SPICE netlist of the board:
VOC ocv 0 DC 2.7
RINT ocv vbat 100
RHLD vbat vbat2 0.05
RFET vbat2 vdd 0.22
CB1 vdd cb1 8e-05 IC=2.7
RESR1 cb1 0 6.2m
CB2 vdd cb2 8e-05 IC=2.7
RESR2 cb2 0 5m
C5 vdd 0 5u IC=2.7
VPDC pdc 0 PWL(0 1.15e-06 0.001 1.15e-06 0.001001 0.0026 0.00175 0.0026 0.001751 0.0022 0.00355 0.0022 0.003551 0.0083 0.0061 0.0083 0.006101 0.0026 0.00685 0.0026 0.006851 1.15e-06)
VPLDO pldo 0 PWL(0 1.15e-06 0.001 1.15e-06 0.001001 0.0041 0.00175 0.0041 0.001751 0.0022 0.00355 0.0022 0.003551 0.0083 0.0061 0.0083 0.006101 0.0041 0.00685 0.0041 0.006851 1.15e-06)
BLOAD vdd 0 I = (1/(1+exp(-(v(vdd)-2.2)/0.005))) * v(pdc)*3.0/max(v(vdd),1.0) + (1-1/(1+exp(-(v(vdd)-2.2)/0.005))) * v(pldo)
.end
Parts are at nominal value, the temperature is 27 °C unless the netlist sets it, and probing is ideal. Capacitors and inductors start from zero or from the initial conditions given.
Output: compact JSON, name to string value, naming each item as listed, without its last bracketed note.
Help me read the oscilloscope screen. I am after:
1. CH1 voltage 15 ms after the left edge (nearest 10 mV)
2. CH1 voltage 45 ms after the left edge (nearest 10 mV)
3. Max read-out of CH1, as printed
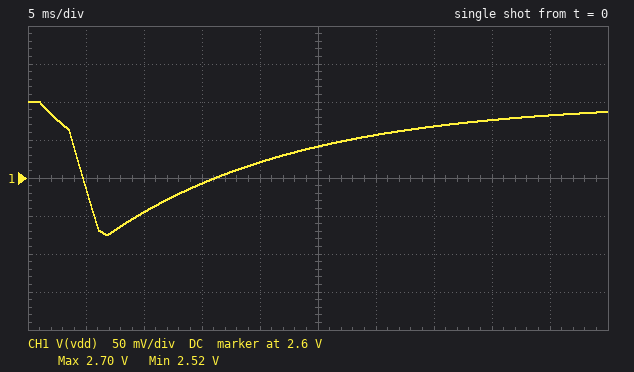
{"CH1 voltage 15 ms after the left edge": "2.59 V", "CH1 voltage 45 ms after the left edge": "2.68 V", "Max read-out of CH1, as printed": "2.70 V"}
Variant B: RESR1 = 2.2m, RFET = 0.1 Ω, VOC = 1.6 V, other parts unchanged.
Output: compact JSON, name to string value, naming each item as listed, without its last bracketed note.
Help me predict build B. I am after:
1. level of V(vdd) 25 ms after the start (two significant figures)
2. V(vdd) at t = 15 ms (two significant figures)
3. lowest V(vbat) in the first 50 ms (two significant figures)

{"level of V(vdd) 25 ms after the start": "1.8 V", "V(vdd) at t = 15 ms": "1.9 V", "lowest V(vbat) in the first 50 ms": "1.6 V"}
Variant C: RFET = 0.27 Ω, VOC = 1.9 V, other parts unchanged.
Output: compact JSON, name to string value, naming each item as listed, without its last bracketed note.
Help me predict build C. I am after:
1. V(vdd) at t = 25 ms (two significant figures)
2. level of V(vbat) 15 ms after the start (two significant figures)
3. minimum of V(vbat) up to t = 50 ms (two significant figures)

{"V(vdd) at t = 25 ms": "2.0 V", "level of V(vbat) 15 ms after the start": "2.1 V", "minimum of V(vbat) up to t = 50 ms": "1.9 V"}
